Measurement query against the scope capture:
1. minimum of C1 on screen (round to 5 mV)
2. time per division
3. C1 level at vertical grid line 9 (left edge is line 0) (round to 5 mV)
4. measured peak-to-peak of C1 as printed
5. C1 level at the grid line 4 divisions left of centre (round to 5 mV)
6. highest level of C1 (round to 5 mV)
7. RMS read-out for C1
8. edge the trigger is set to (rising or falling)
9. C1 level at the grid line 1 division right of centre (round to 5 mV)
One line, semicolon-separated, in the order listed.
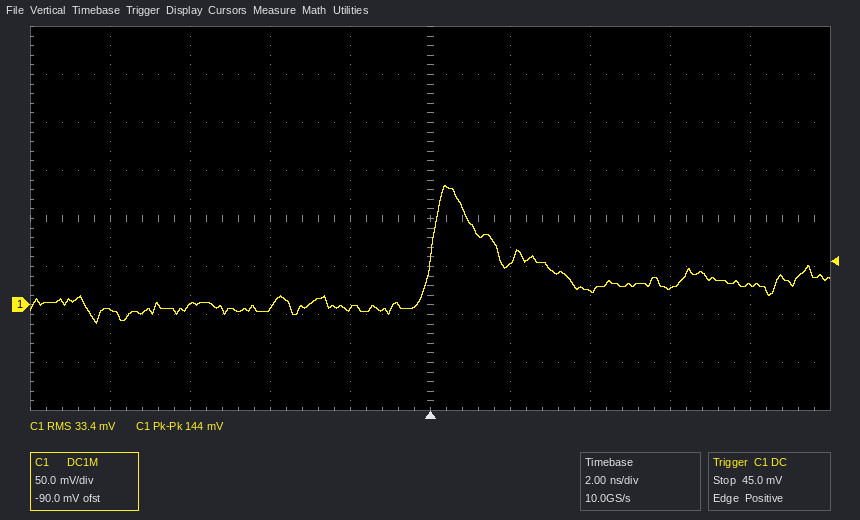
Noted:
-20 mV; 2 ns; 20 mV; 144 mV; -5 mV; 125 mV; 33.4 mV; rising; 45 mV
